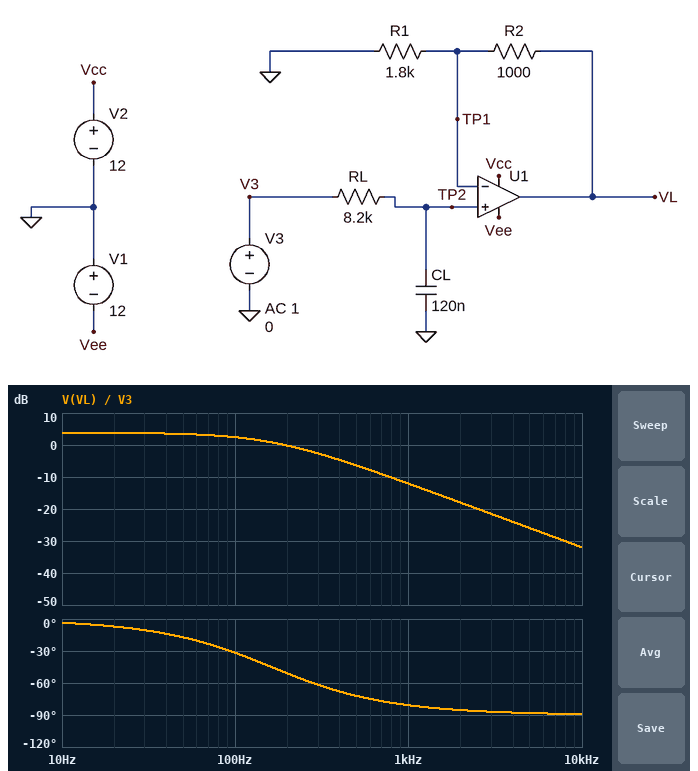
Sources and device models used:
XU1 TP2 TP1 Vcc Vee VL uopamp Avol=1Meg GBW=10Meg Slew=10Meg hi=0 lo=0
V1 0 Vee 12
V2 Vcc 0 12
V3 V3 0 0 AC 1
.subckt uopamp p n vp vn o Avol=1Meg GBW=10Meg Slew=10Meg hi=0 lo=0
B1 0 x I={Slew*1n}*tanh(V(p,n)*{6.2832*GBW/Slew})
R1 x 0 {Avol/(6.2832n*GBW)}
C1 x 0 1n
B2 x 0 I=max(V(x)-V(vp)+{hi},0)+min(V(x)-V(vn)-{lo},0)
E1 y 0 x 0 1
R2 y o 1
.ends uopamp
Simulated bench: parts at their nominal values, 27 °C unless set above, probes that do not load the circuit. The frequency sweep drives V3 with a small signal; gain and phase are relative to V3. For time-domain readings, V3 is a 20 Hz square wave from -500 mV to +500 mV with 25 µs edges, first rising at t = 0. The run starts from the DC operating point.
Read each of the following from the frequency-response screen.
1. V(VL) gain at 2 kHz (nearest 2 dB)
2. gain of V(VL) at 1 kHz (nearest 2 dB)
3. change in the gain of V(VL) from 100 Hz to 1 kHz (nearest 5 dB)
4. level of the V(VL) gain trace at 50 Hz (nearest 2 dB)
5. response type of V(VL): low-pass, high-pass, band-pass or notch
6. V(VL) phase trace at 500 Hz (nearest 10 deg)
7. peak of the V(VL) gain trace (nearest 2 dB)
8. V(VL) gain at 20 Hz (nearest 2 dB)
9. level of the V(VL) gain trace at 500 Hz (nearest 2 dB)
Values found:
-18 dB
-12 dB
-15 dB
4 dB
low-pass
-70 deg
4 dB
4 dB
-6 dB
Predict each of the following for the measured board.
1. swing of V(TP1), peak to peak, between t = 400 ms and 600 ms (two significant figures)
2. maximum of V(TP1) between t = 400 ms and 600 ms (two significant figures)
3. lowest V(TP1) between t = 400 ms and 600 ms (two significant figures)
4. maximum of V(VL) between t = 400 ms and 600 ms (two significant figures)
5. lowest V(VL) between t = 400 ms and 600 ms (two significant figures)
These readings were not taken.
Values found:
1.0 V
500 mV
-500 mV
780 mV
-780 mV
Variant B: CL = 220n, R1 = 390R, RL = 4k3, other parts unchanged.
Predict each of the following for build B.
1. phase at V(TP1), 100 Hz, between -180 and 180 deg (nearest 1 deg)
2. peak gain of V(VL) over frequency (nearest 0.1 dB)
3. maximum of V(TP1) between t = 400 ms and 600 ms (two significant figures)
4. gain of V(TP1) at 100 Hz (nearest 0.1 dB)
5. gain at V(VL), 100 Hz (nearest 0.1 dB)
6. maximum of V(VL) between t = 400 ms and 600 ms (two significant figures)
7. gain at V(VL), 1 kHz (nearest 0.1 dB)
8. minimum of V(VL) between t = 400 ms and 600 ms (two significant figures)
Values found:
-31 deg
11.0 dB
500 mV
-1.3 dB
9.7 dB
1.8 V
-4.6 dB
-1.8 V
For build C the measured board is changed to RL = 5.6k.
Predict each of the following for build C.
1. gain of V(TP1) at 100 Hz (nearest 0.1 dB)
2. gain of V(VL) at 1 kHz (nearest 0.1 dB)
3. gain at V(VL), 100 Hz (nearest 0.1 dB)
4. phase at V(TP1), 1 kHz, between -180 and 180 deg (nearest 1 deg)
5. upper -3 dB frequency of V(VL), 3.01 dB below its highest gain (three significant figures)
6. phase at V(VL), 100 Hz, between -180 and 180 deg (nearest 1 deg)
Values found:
-0.7 dB
-8.9 dB
3.1 dB
-77 deg
237 Hz
-23 deg
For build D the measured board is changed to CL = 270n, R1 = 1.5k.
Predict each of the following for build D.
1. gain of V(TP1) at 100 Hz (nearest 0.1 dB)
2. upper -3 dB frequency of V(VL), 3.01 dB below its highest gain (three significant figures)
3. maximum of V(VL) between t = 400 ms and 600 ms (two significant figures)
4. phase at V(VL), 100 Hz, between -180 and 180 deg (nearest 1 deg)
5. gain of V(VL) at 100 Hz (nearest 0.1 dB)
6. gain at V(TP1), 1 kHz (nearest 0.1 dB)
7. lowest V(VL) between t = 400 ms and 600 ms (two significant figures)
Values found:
-4.7 dB
71.9 Hz
830 mV
-54 deg
-0.2 dB
-22.9 dB
-830 mV
